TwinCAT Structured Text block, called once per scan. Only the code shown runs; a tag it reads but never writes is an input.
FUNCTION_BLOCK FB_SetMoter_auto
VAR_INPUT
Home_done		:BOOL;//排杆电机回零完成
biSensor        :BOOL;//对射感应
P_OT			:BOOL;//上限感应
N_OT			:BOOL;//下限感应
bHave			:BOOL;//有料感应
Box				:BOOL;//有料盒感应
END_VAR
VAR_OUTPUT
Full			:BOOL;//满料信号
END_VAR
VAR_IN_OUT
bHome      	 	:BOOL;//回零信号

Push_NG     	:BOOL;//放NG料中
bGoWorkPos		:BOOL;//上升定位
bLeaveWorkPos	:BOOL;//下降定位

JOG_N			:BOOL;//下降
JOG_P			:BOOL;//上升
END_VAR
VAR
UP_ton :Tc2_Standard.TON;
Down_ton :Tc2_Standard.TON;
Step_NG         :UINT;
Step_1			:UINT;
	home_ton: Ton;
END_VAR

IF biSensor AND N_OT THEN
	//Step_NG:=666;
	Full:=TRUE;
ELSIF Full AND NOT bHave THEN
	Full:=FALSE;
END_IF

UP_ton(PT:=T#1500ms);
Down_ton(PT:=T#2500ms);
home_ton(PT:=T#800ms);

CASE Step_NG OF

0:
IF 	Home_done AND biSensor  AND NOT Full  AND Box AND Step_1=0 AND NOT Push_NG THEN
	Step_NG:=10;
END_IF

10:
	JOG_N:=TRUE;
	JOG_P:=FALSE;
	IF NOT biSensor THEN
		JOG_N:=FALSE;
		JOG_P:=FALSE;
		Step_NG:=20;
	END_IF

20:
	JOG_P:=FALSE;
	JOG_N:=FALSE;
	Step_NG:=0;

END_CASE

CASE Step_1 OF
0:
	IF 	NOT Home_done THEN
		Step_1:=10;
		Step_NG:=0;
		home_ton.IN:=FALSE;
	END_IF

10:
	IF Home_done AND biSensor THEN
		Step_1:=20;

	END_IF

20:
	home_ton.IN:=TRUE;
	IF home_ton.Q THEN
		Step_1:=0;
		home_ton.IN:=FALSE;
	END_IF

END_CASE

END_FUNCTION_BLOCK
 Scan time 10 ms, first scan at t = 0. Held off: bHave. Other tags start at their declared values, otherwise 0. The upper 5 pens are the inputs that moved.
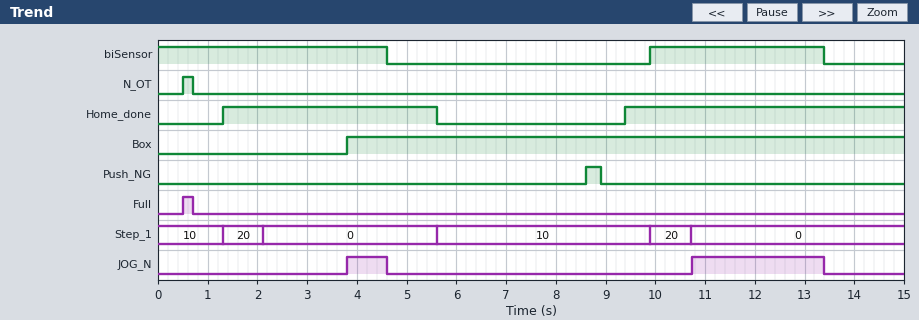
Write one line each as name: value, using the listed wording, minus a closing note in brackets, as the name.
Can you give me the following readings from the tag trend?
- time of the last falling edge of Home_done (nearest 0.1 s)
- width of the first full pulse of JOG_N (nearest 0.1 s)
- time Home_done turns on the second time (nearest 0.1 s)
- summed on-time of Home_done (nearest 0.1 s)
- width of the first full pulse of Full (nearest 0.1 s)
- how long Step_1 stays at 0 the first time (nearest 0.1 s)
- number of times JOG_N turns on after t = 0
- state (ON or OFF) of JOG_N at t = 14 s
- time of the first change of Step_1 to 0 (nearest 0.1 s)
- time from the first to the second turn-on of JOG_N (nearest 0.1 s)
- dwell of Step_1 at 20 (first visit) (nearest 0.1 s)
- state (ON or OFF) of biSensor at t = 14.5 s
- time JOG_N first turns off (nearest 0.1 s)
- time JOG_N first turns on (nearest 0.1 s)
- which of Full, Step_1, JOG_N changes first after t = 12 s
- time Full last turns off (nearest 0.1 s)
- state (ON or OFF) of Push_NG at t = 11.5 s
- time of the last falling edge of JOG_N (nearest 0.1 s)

time of the last falling edge of Home_done: 5.6 s
width of the first full pulse of JOG_N: 0.8 s
time Home_done turns on the second time: 9.4 s
summed on-time of Home_done: 9.9 s
width of the first full pulse of Full: 0.2 s
how long Step_1 stays at 0 the first time: 3.5 s
number of times JOG_N turns on after t = 0: 2
state (ON or OFF) of JOG_N at t = 14 s: OFF
time of the first change of Step_1 to 0: 2.1 s
time from the first to the second turn-on of JOG_N: 6.9 s
dwell of Step_1 at 20 (first visit): 0.8 s
state (ON or OFF) of biSensor at t = 14.5 s: OFF
time JOG_N first turns off: 4.6 s
time JOG_N first turns on: 3.8 s
which of Full, Step_1, JOG_N changes first after t = 12 s: JOG_N
time Full last turns off: 0.7 s
state (ON or OFF) of Push_NG at t = 11.5 s: OFF
time of the last falling edge of JOG_N: 13.4 s
